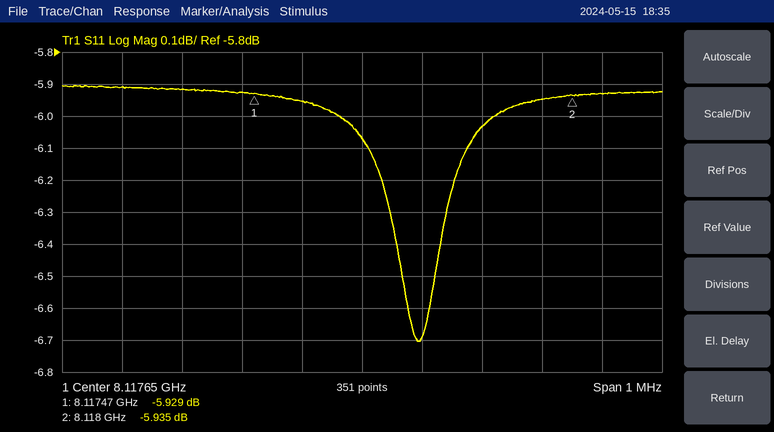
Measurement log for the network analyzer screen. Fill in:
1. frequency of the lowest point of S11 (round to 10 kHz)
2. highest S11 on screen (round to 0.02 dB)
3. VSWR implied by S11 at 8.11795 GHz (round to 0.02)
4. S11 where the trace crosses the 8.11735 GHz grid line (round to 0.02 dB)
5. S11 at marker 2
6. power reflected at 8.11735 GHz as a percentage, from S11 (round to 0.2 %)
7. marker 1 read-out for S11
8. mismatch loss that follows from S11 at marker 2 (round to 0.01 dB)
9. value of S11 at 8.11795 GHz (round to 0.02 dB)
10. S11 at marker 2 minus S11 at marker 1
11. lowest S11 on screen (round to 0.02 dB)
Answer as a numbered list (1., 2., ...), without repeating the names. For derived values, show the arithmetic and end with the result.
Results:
1. 8.11774 GHz
2. -5.90 dB
3. |Γ| = 10^(-5.94/20) = 0.5047; VSWR = (1 + 0.5047)/(1 − 0.5047) ≈ 3.04
4. -5.92 dB
5. -5.935 dB
6. 10^(-5.92/10) ≈ 25.6 %
7. -5.929 dB
8. −10 log10(1 − 10^(-5.935/10)) ≈ 1.28 dB
9. -5.94 dB
10. -5.935 − (-5.929) = -0.006 dB
11. -6.70 dB
